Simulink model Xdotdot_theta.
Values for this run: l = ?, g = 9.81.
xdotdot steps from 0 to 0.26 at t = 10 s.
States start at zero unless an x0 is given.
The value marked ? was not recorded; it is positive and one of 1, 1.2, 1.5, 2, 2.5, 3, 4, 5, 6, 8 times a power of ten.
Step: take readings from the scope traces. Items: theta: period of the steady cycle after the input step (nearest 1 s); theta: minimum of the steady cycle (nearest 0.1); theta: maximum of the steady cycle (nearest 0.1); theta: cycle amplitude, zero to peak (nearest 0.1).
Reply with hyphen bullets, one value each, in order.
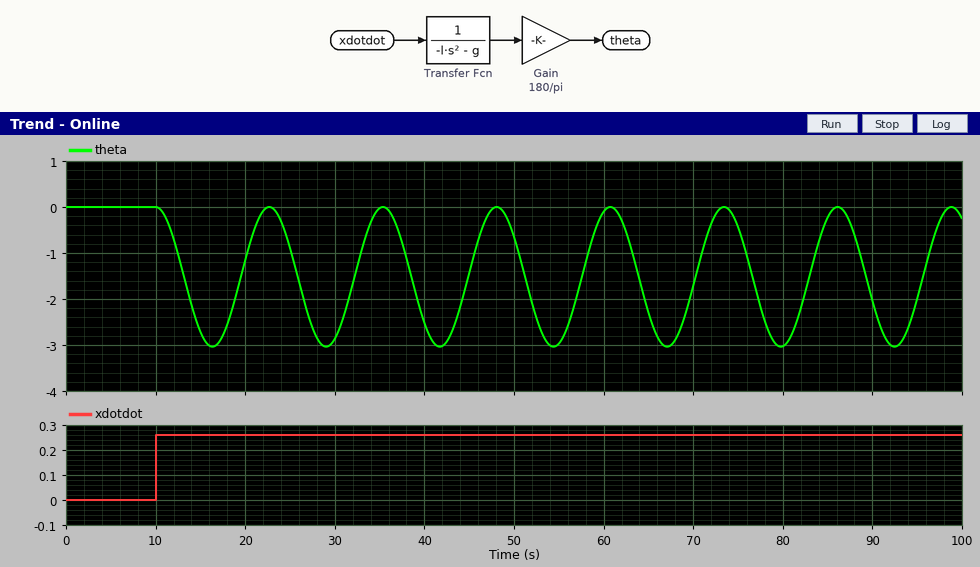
- 13 s
- -3.0
- 0.0
- 1.5
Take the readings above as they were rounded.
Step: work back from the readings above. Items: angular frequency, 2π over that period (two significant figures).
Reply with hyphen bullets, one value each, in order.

- 0.48 rad/s
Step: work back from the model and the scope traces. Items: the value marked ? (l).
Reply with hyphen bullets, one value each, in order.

- 40
